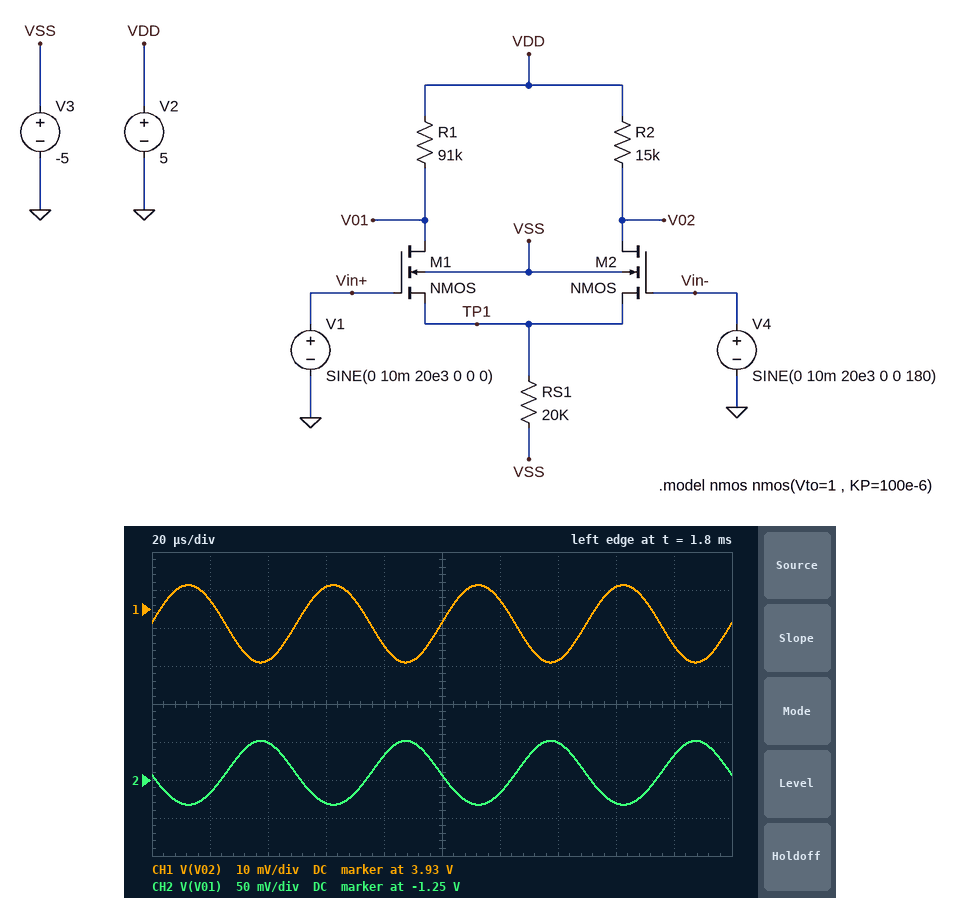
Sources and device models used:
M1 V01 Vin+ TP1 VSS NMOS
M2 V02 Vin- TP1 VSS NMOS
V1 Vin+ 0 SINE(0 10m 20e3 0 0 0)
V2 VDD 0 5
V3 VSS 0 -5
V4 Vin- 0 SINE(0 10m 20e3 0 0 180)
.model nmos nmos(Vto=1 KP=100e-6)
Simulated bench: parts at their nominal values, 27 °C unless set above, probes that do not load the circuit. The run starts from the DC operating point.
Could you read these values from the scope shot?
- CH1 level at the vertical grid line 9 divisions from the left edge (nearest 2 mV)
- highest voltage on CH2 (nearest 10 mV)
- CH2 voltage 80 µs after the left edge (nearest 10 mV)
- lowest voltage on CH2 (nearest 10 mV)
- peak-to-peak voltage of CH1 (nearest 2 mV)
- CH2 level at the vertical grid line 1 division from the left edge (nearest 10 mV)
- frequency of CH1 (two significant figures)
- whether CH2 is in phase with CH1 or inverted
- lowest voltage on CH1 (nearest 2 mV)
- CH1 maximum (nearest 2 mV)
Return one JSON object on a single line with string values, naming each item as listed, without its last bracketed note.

{"CH1 level at the vertical grid line 9 divisions from the left edge": "3.920 V", "highest voltage on CH2": "-1.20 V", "CH2 voltage 80 µs after the left edge": "-1.22 V", "lowest voltage on CH2": "-1.28 V", "peak-to-peak voltage of CH1": "20 mV", "CH2 level at the vertical grid line 1 division from the left edge": "-1.27 V", "frequency of CH1": "20 kHz", "whether CH2 is in phase with CH1 or inverted": "inverted", "lowest voltage on CH1": "3.916 V", "CH1 maximum": "3.936 V"}
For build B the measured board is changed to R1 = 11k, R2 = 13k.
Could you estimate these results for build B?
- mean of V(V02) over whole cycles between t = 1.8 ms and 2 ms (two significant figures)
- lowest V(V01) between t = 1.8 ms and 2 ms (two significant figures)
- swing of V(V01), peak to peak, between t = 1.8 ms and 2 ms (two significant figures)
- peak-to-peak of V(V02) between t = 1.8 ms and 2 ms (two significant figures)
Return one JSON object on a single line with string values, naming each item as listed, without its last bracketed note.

{"mean of V(V02) over whole cycles between t = 1.8 ms and 2 ms": "4.1 V", "lowest V(V01) between t = 1.8 ms and 2 ms": "4.2 V", "swing of V(V01), peak to peak, between t = 1.8 ms and 2 ms": "26 mV", "peak-to-peak of V(V02) between t = 1.8 ms and 2 ms": "31 mV"}
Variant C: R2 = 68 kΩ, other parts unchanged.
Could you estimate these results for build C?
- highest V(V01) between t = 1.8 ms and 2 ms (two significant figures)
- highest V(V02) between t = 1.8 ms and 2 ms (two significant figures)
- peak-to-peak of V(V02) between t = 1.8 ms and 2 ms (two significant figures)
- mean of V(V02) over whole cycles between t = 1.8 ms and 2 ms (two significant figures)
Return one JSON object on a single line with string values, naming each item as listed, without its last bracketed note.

{"highest V(V01) between t = 1.8 ms and 2 ms": "-1.2 V", "highest V(V02) between t = 1.8 ms and 2 ms": "180 mV", "peak-to-peak of V(V02) between t = 1.8 ms and 2 ms": "92 mV", "mean of V(V02) over whole cycles between t = 1.8 ms and 2 ms": "130 mV"}
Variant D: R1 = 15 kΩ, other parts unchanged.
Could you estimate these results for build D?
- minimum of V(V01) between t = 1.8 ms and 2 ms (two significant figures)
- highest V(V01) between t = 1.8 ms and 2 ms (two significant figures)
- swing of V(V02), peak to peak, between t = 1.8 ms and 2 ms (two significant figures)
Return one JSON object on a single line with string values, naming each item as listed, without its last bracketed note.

{"minimum of V(V01) between t = 1.8 ms and 2 ms": "3.9 V", "highest V(V01) between t = 1.8 ms and 2 ms": "4.0 V", "swing of V(V02), peak to peak, between t = 1.8 ms and 2 ms": "36 mV"}
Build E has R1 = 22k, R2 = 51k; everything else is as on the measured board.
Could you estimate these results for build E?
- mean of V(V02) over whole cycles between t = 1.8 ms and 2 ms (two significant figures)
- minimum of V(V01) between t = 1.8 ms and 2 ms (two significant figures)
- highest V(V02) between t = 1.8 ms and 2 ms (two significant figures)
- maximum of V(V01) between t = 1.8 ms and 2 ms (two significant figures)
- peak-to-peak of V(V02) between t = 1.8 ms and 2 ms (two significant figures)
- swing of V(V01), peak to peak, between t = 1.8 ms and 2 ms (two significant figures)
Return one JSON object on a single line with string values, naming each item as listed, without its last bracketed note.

{"mean of V(V02) over whole cycles between t = 1.8 ms and 2 ms": "1.4 V", "minimum of V(V01) between t = 1.8 ms and 2 ms": "3.4 V", "highest V(V02) between t = 1.8 ms and 2 ms": "1.5 V", "maximum of V(V01) between t = 1.8 ms and 2 ms": "3.5 V", "peak-to-peak of V(V02) between t = 1.8 ms and 2 ms": "120 mV", "swing of V(V01), peak to peak, between t = 1.8 ms and 2 ms": "52 mV"}
